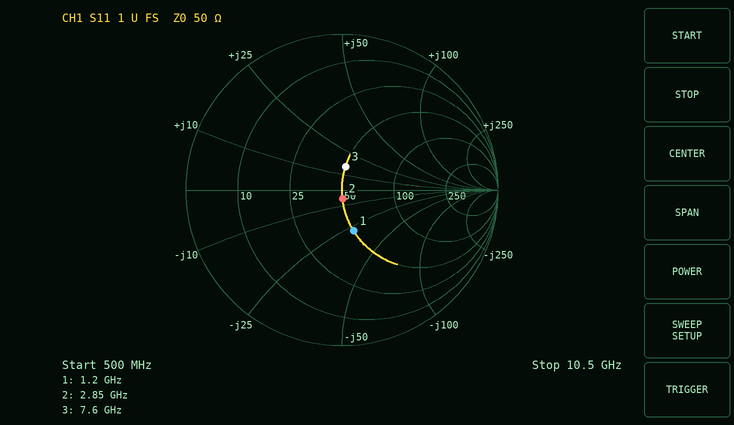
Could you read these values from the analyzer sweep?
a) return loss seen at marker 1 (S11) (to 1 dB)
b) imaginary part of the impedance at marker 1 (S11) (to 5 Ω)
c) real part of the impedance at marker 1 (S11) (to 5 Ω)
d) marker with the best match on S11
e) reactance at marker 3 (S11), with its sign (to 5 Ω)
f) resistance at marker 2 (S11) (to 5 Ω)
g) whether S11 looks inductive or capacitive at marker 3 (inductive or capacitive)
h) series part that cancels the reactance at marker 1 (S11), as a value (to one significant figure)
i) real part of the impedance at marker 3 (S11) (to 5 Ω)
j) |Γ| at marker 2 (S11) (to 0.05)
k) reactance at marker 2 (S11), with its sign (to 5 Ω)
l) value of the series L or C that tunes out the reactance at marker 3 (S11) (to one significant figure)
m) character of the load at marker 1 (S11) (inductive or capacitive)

11 dB
-30 Ω
50 Ω
marker 2
+15 Ω
50 Ω
inductive
4 nH
50 Ω
0.05
-5 Ω
1 pF
capacitive
